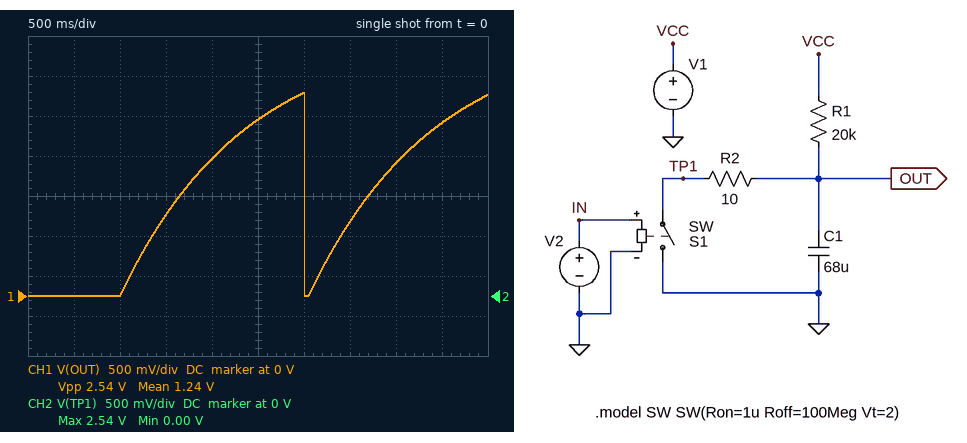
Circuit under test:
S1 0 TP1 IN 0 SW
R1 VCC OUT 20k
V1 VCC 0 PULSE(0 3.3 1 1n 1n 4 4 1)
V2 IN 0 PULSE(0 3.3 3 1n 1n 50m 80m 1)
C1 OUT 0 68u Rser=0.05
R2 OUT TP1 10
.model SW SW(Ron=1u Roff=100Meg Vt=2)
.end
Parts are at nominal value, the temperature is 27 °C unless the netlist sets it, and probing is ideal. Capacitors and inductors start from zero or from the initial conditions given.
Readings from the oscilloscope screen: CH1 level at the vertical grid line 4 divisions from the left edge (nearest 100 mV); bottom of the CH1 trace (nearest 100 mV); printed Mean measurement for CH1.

1.7 V
0 V
1.24 V
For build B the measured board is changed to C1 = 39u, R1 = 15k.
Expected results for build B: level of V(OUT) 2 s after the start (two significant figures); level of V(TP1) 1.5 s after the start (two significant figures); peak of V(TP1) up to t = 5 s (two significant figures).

2.7 V
1.9 V
3.2 V
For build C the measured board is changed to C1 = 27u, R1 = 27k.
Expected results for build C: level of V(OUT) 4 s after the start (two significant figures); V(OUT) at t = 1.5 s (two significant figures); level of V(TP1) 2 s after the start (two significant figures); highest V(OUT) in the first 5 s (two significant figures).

2.4 V
1.6 V
2.5 V
3.1 V
